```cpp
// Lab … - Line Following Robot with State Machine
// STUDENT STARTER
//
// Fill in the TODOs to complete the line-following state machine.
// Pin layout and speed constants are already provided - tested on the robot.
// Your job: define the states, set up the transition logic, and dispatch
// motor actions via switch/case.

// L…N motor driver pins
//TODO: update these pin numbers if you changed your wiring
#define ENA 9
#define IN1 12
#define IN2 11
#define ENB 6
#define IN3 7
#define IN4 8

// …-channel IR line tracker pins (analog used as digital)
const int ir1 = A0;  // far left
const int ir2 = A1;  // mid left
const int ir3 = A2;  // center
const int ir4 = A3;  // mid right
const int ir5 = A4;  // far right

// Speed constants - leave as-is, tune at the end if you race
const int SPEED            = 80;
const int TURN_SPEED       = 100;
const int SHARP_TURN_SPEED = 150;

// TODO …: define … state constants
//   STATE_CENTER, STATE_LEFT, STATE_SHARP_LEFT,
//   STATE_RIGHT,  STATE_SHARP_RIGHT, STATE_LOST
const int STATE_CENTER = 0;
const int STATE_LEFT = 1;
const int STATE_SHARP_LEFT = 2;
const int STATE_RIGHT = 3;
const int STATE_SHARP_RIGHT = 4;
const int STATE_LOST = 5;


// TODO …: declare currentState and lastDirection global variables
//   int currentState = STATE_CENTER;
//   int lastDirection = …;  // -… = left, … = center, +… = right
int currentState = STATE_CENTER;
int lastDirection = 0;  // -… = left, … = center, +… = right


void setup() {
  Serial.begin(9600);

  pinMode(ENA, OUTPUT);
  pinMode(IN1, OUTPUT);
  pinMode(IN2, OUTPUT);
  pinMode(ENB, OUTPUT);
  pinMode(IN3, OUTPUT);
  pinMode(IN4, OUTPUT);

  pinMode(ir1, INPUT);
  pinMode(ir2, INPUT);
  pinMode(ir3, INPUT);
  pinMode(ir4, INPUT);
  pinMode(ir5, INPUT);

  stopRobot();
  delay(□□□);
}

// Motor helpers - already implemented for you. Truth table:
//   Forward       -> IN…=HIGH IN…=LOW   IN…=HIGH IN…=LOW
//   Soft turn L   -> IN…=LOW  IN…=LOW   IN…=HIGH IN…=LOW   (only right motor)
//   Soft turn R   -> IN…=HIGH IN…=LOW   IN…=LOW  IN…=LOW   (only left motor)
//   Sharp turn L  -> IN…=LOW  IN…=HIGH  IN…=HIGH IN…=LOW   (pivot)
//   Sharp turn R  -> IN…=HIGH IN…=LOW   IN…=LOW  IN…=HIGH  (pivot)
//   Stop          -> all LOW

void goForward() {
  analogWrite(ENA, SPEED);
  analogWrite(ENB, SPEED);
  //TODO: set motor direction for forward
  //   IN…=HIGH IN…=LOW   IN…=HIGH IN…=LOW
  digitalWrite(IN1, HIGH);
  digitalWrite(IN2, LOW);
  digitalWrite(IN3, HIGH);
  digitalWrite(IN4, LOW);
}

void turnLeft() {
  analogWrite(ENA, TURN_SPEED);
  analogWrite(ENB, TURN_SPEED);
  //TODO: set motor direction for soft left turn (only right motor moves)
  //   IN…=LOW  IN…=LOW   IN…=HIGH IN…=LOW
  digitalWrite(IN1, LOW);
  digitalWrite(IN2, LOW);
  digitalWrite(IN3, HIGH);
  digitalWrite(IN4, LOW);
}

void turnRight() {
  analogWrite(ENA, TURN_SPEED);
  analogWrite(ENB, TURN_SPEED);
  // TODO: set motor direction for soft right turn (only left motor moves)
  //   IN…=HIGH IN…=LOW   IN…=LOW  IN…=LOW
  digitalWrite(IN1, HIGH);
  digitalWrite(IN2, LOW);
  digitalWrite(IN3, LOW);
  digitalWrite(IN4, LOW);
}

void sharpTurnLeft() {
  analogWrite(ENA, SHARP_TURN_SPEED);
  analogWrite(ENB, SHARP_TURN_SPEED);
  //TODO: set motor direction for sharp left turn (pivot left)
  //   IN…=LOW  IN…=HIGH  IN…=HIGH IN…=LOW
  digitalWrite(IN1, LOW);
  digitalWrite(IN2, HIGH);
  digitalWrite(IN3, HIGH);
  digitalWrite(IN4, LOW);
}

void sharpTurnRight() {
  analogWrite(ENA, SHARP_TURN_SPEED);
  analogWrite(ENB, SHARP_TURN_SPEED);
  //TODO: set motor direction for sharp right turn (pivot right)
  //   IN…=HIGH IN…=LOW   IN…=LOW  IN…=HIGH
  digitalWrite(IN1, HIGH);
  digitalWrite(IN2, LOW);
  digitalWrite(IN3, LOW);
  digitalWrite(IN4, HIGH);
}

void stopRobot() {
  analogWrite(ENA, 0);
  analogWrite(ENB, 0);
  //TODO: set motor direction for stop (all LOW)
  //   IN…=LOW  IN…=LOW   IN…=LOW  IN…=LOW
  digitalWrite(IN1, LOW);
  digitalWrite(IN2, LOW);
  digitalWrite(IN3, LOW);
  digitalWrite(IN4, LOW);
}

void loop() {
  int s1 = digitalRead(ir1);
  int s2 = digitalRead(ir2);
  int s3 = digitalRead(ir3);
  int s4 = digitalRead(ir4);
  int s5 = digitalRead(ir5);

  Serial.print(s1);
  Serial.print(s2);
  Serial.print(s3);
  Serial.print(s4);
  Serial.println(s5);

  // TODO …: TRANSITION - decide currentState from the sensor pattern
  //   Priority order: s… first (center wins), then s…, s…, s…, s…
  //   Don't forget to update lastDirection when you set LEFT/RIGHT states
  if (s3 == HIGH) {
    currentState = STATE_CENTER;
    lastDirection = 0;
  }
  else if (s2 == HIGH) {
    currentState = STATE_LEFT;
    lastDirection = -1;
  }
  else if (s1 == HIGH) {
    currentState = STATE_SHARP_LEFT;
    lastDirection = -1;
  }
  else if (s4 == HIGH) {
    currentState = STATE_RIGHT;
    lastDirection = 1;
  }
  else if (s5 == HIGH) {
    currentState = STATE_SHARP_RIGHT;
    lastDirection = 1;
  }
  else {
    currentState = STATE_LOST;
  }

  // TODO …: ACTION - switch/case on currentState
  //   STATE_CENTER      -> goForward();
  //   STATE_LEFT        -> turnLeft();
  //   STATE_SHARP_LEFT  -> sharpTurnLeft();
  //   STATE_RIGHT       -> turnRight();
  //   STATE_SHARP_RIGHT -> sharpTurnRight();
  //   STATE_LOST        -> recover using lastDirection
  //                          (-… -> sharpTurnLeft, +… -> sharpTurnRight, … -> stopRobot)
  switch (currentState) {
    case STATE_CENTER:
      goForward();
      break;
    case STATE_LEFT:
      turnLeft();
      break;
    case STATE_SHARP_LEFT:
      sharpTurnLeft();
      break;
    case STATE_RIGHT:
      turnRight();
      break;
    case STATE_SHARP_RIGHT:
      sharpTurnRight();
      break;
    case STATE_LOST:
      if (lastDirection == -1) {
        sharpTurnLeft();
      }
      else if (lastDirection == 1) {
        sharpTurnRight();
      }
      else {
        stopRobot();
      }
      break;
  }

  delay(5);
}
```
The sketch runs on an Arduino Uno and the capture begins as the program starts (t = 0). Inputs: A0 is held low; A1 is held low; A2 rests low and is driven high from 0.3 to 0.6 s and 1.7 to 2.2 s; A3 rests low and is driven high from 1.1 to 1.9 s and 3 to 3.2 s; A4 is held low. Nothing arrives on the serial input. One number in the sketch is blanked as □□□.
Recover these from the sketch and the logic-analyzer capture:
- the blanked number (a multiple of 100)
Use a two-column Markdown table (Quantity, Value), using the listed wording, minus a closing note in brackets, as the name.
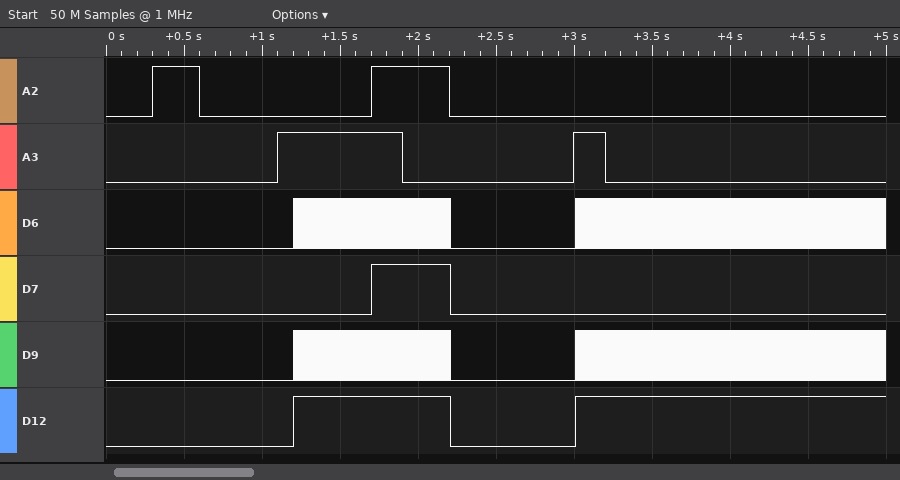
| Quantity | Value |
|---|---|
| the blanked number | 1200 |
